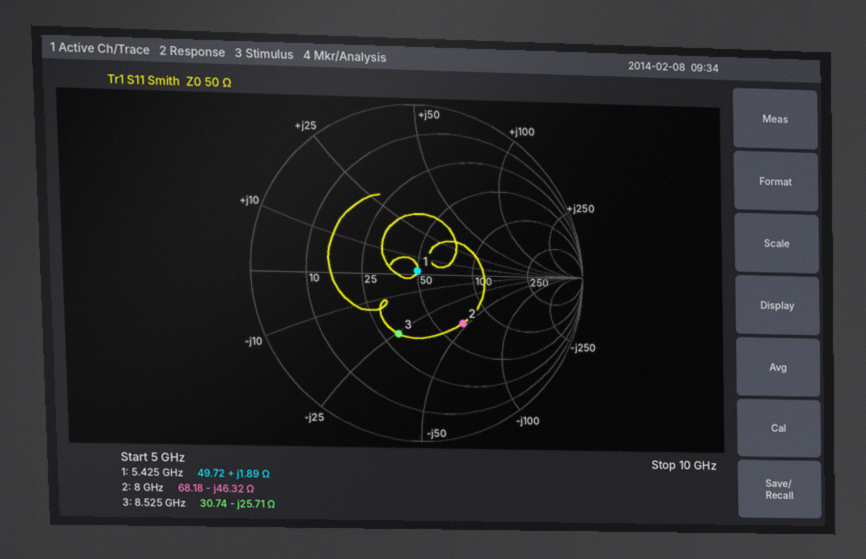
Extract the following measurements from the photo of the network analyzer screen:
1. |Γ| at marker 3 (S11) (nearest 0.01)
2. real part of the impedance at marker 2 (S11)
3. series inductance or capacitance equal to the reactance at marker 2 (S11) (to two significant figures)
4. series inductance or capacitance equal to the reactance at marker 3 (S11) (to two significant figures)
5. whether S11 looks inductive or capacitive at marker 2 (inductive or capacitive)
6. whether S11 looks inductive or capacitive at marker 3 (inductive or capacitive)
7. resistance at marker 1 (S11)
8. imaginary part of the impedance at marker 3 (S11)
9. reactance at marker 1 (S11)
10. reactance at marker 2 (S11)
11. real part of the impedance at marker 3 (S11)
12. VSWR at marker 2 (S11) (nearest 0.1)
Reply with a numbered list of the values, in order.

1. 0.38
2. 68.18 Ω
3. 430 fF
4. 730 fF
5. capacitive
6. capacitive
7. 49.72 Ω
8. -25.71 Ω
9. +1.89 Ω
10. -46.32 Ω
11. 30.74 Ω
12. 2.3
